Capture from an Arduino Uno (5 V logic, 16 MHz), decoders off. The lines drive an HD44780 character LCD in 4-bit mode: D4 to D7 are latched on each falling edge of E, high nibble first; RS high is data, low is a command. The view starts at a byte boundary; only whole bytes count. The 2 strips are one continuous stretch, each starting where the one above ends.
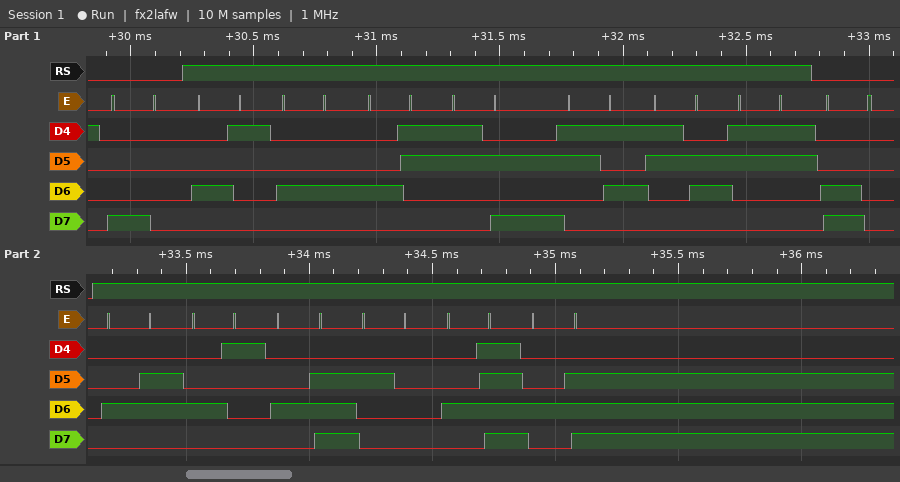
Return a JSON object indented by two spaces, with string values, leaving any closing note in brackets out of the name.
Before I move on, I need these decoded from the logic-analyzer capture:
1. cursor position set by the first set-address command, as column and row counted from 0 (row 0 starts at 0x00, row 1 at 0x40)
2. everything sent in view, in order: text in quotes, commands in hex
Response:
{
  "cursor position set by the first set-address command, as column and row counted from 0": "column 0, row 0",
  "everything sent in view, in order: text in quotes, commands in hex": "0x80 \"ADC:563\" 0xC0 \"FAN ON\""
}
